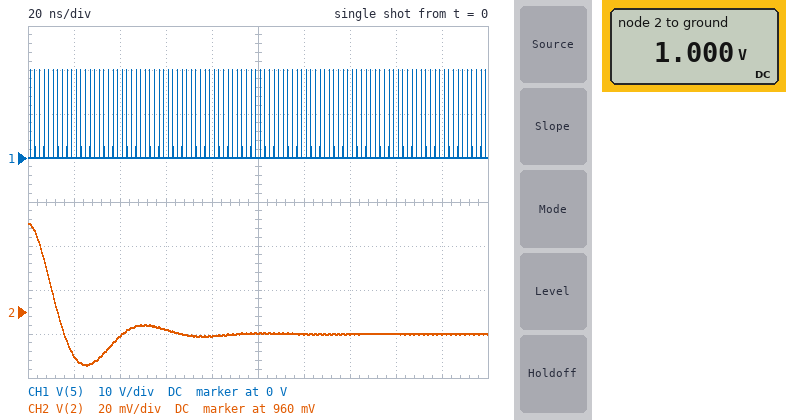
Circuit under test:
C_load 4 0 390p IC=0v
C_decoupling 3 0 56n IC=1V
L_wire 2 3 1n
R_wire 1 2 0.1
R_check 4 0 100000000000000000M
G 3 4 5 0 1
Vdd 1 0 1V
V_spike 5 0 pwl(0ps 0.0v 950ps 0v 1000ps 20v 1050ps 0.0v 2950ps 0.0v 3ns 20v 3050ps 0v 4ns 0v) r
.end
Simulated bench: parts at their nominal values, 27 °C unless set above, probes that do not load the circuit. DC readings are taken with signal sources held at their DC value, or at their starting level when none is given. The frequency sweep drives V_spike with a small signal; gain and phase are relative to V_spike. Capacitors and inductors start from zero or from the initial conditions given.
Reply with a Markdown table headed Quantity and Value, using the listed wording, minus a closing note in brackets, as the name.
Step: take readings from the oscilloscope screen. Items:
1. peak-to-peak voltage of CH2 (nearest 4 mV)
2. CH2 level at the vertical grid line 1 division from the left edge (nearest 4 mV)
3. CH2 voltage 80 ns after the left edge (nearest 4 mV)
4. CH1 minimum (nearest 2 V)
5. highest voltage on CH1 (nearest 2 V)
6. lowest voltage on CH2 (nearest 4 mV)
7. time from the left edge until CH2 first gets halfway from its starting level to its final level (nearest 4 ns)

| Quantity | Value |
|---|---|
| peak-to-peak voltage of CH2 | 64 mV |
| CH2 level at the vertical grid line 1 division from the left edge | 940 mV |
| CH2 voltage 80 ns after the left edge | 948 mV |
| CH1 minimum | 0 V |
| highest voltage on CH1 | 20 V |
| lowest voltage on CH2 | 936 mV |
| time from the left edge until CH2 first gets halfway from its starting level to its final level | 8 ns |
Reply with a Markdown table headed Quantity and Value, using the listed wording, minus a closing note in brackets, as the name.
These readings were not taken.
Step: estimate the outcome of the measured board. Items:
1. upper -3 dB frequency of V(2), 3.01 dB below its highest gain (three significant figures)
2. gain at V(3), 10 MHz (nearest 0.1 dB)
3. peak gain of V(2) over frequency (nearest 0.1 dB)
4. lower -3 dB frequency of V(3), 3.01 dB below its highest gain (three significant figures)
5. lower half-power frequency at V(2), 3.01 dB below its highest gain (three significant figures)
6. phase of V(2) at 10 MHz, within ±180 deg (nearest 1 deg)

| Quantity | Value |
|---|---|
| upper -3 dB frequency of V(2), 3.01 dB below its highest gain | 25.3 MHz |
| gain at V(3), 10 MHz | -17.2 dB |
| peak gain of V(2) over frequency | -16.8 dB |
| lower -3 dB frequency of V(3), 3.01 dB below its highest gain | 12.3 MHz |
| lower half-power frequency at V(2), 3.01 dB below its highest gain | 3.43 MHz |
| phase of V(2) at 10 MHz, within ±180 deg | 156 deg |
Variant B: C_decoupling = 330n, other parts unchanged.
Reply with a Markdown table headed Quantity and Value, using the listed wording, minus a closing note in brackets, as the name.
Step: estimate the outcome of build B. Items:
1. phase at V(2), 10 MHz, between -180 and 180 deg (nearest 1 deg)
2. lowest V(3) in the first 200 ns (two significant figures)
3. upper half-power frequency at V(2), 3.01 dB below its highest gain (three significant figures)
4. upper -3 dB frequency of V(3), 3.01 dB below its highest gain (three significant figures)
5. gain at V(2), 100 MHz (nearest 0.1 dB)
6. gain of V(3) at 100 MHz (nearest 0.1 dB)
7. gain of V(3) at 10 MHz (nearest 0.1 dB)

| Quantity | Value |
|---|---|
| phase at V(2), 10 MHz, between -180 and 180 deg | 82 deg |
| lowest V(3) in the first 200 ns | 950 mV |
| upper half-power frequency at V(2), 3.01 dB below its highest gain | 6.45 MHz |
| upper -3 dB frequency of V(3), 3.01 dB below its highest gain | 7.39 MHz |
| gain at V(2), 100 MHz | -62.3 dB |
| gain of V(3) at 100 MHz | -46.3 dB |
| gain of V(3) at 10 MHz | -25.0 dB |
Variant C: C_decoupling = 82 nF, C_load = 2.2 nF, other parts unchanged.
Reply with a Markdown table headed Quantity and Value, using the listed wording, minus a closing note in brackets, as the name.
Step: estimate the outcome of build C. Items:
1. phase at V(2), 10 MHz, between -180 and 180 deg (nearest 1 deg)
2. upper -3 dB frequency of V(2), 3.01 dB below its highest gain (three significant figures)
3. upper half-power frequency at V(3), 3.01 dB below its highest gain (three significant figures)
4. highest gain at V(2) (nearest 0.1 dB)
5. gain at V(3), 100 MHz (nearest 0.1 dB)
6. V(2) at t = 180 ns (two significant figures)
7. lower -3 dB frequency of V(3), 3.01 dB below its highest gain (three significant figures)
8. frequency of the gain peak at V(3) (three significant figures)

| Quantity | Value |
|---|---|
| phase at V(2), 10 MHz, between -180 and 180 deg | 143 deg |
| upper -3 dB frequency of V(2), 3.01 dB below its highest gain | 20.8 MHz |
| upper half-power frequency at V(3), 3.01 dB below its highest gain | 24.1 MHz |
| highest gain at V(2) | -18.1 dB |
| gain at V(3), 100 MHz | -34.0 dB |
| V(2) at t = 180 ns | 950 mV |
| lower -3 dB frequency of V(3), 3.01 dB below its highest gain | 6.96 MHz |
| frequency of the gain peak at V(3) | 15.8 MHz |
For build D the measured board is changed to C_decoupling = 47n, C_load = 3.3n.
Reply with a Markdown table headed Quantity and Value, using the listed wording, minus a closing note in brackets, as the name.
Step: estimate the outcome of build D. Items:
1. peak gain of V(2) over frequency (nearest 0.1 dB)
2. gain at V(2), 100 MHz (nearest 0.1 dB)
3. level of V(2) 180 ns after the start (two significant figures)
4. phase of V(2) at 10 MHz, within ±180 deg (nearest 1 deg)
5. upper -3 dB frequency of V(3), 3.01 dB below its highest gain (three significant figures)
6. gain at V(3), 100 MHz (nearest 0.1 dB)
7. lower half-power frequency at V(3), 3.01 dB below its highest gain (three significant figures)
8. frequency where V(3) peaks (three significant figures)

| Quantity | Value |
|---|---|
| peak gain of V(2) over frequency | -16.2 dB |
| gain at V(2), 100 MHz | -45.0 dB |
| level of V(2) 180 ns after the start | 950 mV |
| phase of V(2) at 10 MHz, within ±180 deg | 160 deg |
| upper -3 dB frequency of V(3), 3.01 dB below its highest gain | 30.8 MHz |
| gain at V(3), 100 MHz | -28.9 dB |
| lower half-power frequency at V(3), 3.01 dB below its highest gain | 14.7 MHz |
| frequency where V(3) peaks | 22.3 MHz |
